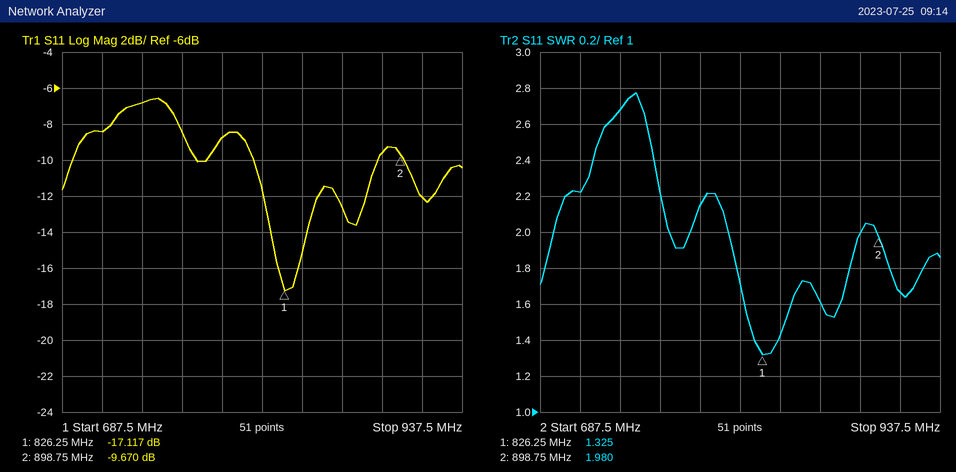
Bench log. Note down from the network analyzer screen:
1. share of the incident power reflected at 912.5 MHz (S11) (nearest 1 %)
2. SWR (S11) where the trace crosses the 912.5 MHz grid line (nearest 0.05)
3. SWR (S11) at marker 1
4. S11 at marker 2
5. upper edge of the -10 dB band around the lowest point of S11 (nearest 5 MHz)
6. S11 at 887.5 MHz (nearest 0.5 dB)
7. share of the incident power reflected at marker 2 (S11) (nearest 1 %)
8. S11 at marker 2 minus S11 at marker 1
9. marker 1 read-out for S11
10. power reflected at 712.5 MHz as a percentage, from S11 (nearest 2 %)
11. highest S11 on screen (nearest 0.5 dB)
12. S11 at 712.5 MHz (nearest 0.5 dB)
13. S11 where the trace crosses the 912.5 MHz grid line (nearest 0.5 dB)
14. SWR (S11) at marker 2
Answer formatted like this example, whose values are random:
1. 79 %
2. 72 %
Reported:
1. 6 %
2. 1.65
3. 1.325
4. -9.670 dB
5. 885 MHz
6. -9.5 dB
7. 11 %
8. 7.447 dB
9. -17.117 dB
10. 14 %
11. -6.5 dB
12. -8.5 dB
13. -12.0 dB
14. 1.980
